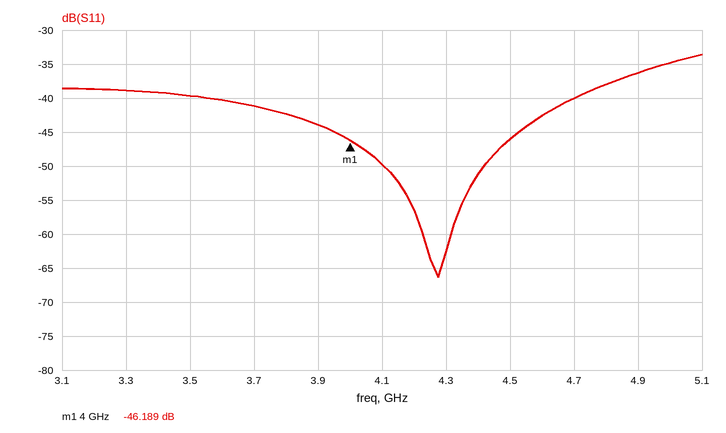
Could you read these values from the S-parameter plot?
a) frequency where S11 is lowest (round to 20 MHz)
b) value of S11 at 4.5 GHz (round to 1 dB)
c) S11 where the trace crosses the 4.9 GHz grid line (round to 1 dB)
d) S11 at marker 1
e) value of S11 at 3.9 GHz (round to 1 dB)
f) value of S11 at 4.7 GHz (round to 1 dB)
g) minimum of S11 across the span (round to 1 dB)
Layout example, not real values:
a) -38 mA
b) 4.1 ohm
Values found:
a) 4.28 GHz
b) -46 dB
c) -36 dB
d) -46.189 dB
e) -44 dB
f) -40 dB
g) -66 dB
